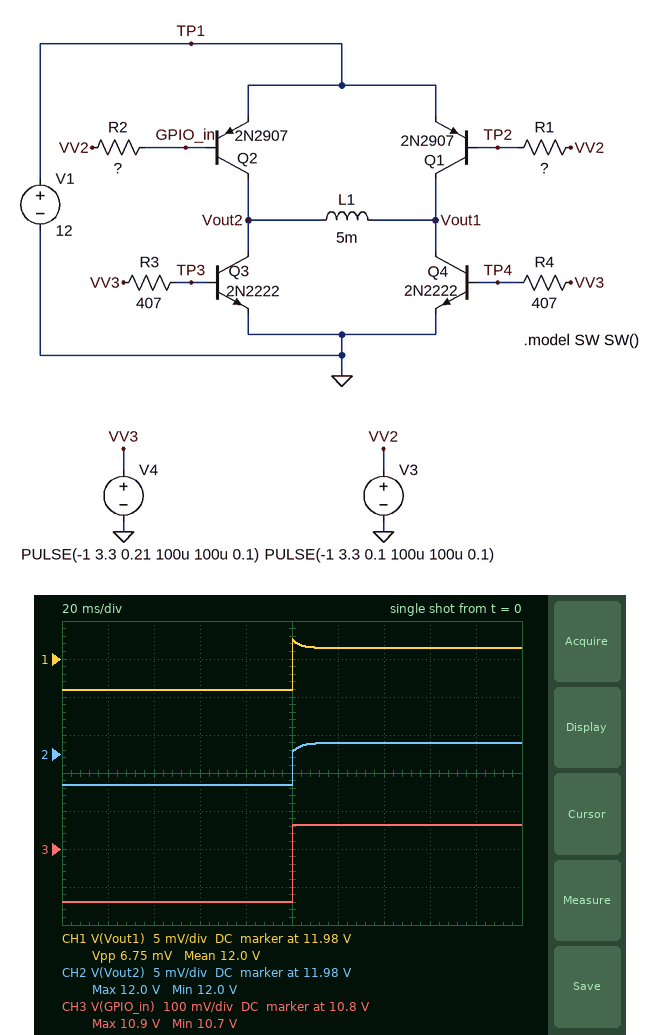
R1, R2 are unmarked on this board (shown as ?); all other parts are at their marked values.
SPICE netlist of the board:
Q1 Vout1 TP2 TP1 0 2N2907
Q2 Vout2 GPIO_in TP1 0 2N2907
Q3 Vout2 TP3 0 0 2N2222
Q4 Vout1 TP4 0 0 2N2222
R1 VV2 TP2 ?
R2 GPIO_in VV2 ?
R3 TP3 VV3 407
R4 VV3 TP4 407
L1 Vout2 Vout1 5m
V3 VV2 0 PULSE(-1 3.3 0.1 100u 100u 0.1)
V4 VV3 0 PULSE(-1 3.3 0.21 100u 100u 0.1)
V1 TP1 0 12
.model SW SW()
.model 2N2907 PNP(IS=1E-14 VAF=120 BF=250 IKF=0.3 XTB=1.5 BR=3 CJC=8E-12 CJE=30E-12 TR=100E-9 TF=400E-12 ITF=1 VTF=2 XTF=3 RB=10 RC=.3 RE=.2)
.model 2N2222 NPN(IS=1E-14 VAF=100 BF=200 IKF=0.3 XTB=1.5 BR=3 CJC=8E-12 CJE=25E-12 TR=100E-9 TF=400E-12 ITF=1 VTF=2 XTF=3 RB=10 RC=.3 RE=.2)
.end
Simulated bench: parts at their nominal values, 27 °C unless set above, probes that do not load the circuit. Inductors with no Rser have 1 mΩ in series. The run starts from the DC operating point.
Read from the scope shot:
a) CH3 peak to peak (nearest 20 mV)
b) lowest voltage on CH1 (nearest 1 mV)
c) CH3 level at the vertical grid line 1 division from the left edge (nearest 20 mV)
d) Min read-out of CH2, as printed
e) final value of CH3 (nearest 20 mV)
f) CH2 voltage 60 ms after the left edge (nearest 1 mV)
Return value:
200 mV
11.976 V
10.66 V
12.0 V
10.86 V
11.976 V
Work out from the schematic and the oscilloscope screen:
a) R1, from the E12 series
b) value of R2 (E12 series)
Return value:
150 Ω
220 Ω
